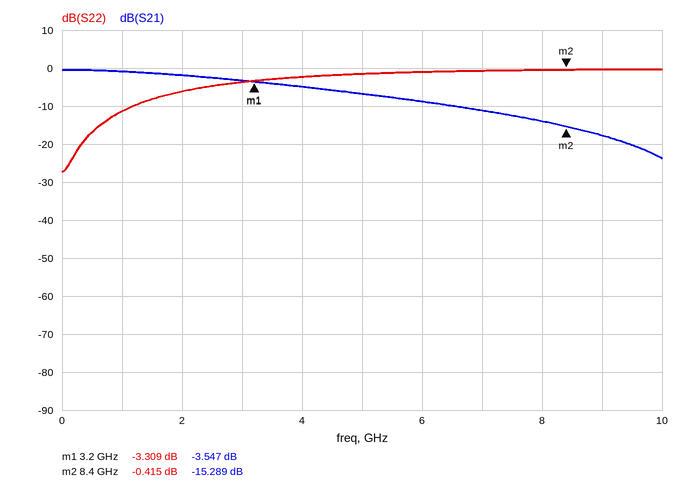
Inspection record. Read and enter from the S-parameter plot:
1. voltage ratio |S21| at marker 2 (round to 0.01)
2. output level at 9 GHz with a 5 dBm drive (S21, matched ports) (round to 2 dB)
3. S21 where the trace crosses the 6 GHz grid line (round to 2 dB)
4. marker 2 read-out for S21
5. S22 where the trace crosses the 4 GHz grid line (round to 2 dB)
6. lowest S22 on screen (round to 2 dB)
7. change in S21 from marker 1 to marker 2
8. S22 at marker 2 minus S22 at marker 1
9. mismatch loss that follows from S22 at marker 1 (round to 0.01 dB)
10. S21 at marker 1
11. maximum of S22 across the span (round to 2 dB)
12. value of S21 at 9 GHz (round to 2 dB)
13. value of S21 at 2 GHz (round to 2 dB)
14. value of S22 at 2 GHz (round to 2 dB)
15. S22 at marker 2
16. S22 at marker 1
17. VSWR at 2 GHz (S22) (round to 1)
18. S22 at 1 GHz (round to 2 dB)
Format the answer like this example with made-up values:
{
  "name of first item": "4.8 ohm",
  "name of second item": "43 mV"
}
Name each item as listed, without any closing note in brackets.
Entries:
{
  "voltage ratio |S21| at marker 2": "0.17",
  "output level at 9 GHz with a 5 dBm drive (S21, matched ports)": "-12 dBm",
  "S21 where the trace crosses the 6 GHz grid line": "-8 dB",
  "marker 2 read-out for S21": "-15.289 dB",
  "S22 where the trace crosses the 4 GHz grid line": "-2 dB",
  "lowest S22 on screen": "-28 dB",
  "change in S21 from marker 1 to marker 2": "-11.742 dB",
  "S22 at marker 2 minus S22 at marker 1": "2.894 dB",
  "mismatch loss that follows from S22 at marker 1": "2.73 dB",
  "S21 at marker 1": "-3.547 dB",
  "maximum of S22 across the span": "0 dB",
  "value of S21 at 9 GHz": "-18 dB",
  "value of S21 at 2 GHz": "-2 dB",
  "value of S22 at 2 GHz": "-6 dB",
  "S22 at marker 2": "-0.415 dB",
  "S22 at marker 1": "-3.309 dB",
  "VSWR at 2 GHz (S22)": "3",
  "S22 at 1 GHz": "-12 dB"
}
